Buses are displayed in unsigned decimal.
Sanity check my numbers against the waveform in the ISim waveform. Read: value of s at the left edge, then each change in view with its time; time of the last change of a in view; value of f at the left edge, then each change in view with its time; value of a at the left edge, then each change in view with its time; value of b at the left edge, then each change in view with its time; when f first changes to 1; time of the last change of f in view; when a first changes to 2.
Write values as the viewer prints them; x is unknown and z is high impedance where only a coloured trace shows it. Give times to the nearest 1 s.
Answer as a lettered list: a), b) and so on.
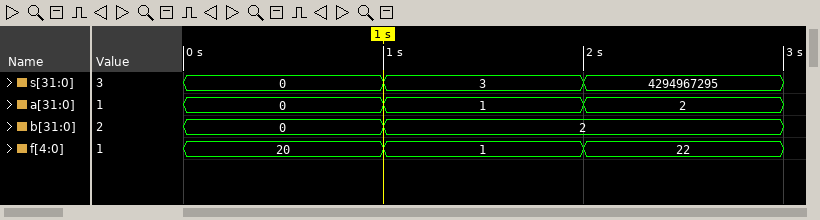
a) 0, 3 at 1 s, 4294967295 at 2 s
b) 2 s
c) 20, 1 at 1 s, 22 at 2 s
d) 0, 1 at 1 s, 2 at 2 s
e) 0, 2 at 1 s
f) 1 s
g) 2 s
h) 2 s
